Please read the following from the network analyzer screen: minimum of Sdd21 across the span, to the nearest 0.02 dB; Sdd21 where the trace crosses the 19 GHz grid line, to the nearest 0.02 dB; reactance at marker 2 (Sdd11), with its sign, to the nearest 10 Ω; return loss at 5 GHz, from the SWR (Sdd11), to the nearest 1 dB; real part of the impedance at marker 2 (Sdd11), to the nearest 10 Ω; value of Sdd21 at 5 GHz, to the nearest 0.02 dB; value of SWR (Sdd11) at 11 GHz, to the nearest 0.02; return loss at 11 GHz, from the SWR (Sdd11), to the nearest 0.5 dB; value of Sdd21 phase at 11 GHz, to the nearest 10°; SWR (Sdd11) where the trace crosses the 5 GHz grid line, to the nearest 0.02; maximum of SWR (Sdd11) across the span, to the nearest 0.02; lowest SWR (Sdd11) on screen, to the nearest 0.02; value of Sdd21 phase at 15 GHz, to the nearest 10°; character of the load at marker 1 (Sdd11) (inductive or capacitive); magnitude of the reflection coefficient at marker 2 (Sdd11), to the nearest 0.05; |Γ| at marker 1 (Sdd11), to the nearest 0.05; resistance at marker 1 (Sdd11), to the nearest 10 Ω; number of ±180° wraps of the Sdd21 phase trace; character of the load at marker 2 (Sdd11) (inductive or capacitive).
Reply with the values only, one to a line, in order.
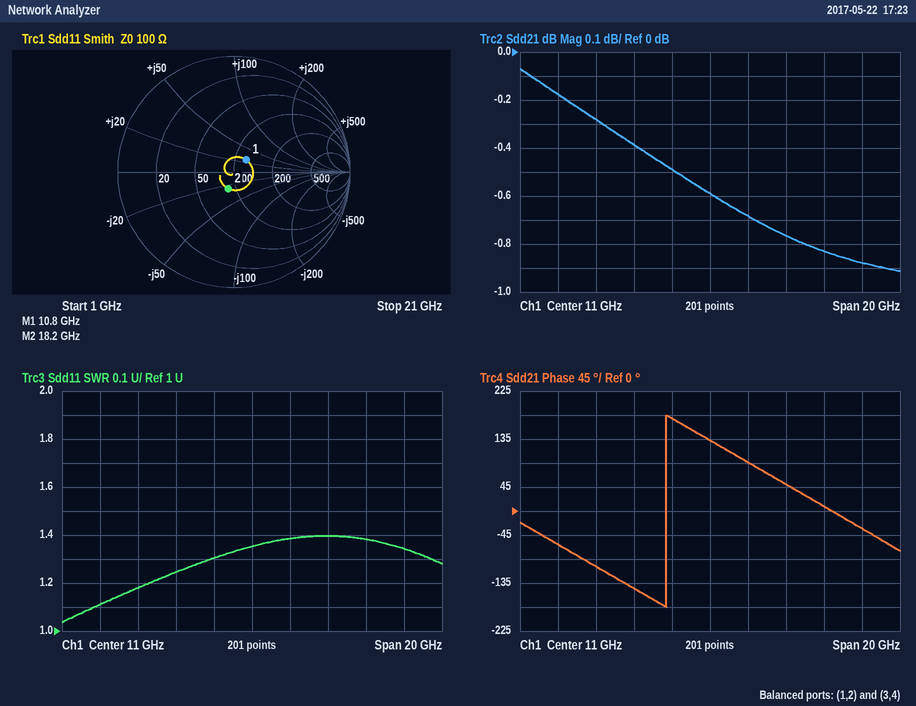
-0.92 dB
-0.88 dB
-30 Ω
22 dB
90 Ω
-0.28 dB
1.36
16.5 dB
130°
1.18
1.40
1.04
50°
inductive
0.15
0.15
120 Ω
1
capacitive
